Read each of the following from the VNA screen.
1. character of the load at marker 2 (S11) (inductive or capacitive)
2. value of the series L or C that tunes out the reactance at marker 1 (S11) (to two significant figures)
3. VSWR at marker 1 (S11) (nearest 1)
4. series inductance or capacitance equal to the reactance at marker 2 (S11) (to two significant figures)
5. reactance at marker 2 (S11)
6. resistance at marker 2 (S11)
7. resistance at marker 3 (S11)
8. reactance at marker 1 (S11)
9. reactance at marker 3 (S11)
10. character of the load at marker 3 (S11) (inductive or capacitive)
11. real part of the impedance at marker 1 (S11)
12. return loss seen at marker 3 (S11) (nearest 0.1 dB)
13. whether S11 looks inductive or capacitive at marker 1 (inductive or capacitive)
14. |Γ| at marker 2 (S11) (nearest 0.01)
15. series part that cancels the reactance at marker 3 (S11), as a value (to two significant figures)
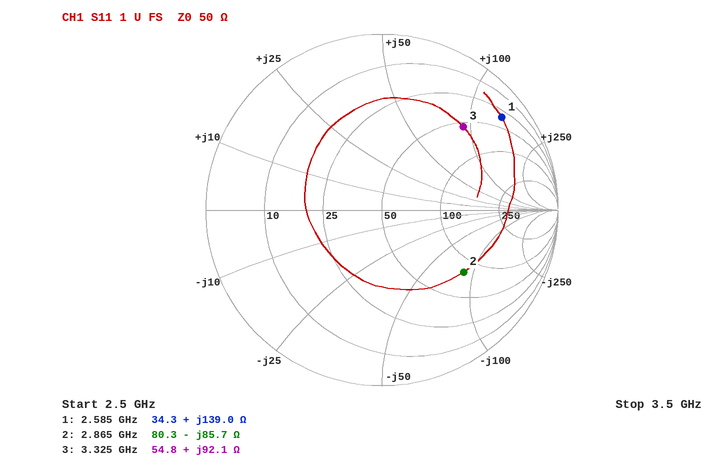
capacitive
440 fF
13
650 fF
-85.7 Ω
80.3 Ω
54.8 Ω
+139.0 Ω
+92.1 Ω
inductive
34.3 Ω
3.6 dB
inductive
0.58
520 fF
